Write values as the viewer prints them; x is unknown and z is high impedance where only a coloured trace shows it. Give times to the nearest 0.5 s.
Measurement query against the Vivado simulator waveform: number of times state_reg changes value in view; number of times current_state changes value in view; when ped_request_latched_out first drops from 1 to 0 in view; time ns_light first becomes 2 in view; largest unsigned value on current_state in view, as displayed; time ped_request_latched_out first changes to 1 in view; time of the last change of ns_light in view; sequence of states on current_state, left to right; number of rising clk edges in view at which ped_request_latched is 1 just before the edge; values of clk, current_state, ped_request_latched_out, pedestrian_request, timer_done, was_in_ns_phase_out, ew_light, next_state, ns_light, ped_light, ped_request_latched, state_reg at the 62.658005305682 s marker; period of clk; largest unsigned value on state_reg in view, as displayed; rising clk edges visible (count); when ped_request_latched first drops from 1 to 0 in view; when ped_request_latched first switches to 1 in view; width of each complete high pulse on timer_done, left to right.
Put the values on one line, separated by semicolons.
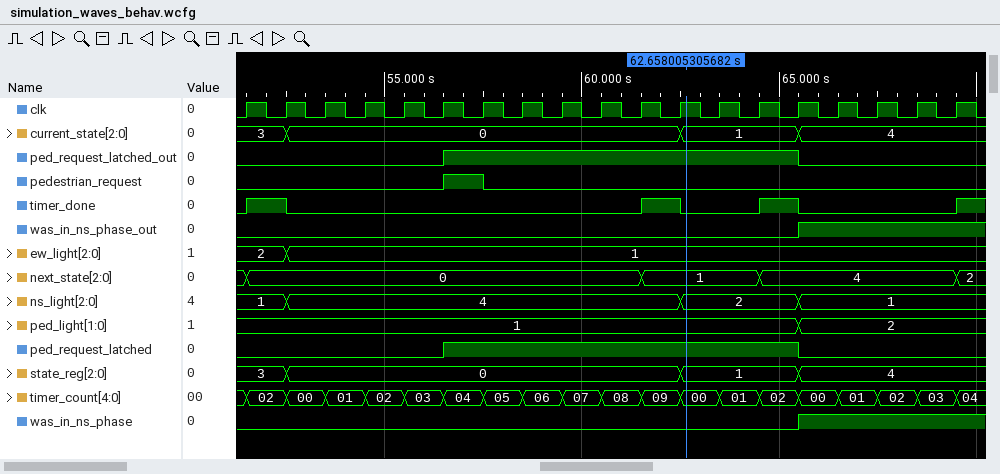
3; 3; 65.5 s; 62.5 s; 4; 56.5 s; 65.5 s; 3, 0, 1, 4; 9; clk=1, current_state=1, ped_request_latched_out=1, pedestrian_request=0, timer_done=0, was_in_ns_phase_out=0, ew_light=1, next_state=1, ns_light=2, ped_light=1, ped_request_latched=1, state_reg=1; 1 s; 4; 19; 65.5 s; 56.5 s; 1 s, 1 s, 1 s
